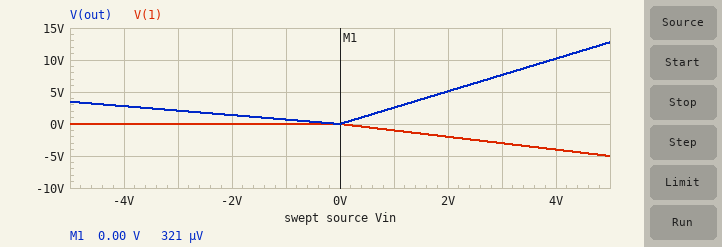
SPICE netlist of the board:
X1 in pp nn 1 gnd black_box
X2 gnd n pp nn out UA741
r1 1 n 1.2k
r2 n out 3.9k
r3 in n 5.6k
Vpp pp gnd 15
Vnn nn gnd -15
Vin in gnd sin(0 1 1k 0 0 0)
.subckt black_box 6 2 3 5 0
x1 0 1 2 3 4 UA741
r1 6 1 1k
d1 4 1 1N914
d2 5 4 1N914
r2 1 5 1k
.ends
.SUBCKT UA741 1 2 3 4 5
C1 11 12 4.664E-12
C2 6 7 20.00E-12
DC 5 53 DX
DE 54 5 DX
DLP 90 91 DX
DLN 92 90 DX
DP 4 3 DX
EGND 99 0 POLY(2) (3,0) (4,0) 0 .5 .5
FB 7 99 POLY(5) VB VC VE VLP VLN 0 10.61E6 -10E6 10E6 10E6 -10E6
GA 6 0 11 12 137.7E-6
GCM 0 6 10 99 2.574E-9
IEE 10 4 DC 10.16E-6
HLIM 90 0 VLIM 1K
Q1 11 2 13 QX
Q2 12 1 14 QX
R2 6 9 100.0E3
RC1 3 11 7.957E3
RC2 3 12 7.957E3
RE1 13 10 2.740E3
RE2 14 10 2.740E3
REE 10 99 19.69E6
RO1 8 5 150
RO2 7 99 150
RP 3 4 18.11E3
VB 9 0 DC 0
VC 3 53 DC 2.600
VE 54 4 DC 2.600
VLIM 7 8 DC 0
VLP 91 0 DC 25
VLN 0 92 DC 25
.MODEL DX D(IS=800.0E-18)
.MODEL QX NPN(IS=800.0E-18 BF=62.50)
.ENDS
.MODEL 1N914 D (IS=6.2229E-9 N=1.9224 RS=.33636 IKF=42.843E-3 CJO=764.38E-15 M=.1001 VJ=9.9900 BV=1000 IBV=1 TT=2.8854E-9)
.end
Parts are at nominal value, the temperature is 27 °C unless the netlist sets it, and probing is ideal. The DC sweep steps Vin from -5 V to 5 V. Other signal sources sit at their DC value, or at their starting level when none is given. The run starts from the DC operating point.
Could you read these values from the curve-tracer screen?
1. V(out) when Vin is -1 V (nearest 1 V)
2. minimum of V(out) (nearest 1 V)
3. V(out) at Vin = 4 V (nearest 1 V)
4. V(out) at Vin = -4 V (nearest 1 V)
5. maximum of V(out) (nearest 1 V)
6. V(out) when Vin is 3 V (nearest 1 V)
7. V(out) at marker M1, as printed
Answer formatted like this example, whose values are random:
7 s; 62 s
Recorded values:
1 V; 0 V; 10 V; 3 V; 13 V; 8 V; 321 µV
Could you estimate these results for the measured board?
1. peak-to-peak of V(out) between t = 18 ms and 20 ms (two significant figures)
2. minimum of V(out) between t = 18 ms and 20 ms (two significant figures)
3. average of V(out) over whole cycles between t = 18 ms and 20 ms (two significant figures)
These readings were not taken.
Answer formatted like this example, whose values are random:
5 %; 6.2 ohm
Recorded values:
2.6 V; -69 mV; 1.0 V
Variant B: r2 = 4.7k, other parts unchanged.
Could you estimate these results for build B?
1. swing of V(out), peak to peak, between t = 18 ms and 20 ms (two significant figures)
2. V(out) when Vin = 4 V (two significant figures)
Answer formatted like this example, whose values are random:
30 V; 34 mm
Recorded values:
3.2 V; 12 V
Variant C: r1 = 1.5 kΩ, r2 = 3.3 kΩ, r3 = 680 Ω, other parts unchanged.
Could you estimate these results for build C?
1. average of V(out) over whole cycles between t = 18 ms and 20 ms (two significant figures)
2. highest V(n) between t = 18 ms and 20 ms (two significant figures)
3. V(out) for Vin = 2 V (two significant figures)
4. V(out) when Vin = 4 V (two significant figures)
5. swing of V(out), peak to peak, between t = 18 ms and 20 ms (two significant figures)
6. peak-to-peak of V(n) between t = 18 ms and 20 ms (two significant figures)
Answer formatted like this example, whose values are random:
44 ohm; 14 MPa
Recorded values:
700 mV; 5.5 mV; -5.3 V; -11 V; 7.5 V; 11 mV
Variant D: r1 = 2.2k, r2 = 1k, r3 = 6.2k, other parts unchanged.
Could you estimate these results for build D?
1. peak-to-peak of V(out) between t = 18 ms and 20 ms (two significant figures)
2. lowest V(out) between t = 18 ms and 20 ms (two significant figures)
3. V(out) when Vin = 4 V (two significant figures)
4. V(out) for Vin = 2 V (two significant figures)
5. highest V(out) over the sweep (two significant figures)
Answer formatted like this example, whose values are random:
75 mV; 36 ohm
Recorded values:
310 mV; -14 mV; 1.2 V; 590 mV; 1.5 V
